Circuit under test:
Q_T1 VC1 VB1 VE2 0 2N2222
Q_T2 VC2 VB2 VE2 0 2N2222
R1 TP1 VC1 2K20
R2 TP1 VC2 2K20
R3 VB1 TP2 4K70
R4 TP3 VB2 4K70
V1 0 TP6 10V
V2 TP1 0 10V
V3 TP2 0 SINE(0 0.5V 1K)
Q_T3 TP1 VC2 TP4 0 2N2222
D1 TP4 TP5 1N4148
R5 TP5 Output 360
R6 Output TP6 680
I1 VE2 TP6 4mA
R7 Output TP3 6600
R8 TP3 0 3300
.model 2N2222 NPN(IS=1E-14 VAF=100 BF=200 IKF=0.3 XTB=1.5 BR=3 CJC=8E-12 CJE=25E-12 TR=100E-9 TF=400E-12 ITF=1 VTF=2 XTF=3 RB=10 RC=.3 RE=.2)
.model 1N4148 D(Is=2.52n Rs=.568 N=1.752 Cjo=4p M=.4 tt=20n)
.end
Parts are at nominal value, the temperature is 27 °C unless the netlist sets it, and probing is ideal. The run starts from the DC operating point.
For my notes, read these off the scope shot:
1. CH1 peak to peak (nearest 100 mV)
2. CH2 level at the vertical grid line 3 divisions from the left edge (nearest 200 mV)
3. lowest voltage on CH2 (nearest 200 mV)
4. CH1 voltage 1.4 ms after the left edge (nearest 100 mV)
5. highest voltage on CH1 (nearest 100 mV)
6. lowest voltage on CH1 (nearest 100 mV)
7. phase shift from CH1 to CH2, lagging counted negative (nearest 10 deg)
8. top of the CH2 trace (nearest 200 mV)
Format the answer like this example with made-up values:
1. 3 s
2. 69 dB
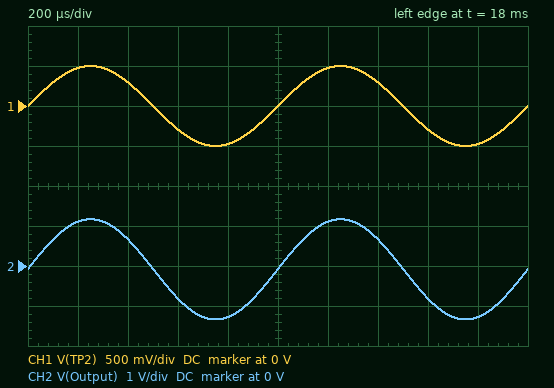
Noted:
1. 1.0 V
2. -800 mV
3. -1.4 V
4. 300 mV
5. 500 mV
6. -500 mV
7. 0 deg
8. 1.2 V
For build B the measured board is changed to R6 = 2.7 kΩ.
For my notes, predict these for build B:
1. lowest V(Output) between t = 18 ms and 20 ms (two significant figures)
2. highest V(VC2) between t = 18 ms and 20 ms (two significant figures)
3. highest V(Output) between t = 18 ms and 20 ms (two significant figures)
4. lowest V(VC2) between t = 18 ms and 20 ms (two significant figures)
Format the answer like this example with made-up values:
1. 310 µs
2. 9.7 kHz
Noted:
1. -880 mV
2. 4.6 V
3. 1.7 V
4. 1.6 V
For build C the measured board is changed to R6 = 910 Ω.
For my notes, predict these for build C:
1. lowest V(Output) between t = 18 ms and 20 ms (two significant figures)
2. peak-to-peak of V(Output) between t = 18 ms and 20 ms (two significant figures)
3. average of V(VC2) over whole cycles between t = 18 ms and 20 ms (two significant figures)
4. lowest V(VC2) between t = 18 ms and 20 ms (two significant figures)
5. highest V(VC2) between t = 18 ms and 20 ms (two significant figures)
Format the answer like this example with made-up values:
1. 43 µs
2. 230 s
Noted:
1. -1.2 V
2. 2.6 V
3. 5.5 V
4. 3.6 V
5. 7.3 V
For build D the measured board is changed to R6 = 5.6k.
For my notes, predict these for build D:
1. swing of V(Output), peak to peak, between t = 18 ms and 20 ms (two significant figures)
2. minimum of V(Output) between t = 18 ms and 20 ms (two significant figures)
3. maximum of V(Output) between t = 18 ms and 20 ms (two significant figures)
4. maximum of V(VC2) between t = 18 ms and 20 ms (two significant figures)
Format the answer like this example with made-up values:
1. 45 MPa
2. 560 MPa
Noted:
1. 2.4 V
2. -610 mV
3. 1.8 V
4. 3.9 V
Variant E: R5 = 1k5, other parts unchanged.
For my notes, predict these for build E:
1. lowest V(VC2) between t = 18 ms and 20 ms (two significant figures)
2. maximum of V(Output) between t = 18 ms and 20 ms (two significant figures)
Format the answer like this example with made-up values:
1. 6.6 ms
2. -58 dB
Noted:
1. 9.9 V
2. -4.0 V
